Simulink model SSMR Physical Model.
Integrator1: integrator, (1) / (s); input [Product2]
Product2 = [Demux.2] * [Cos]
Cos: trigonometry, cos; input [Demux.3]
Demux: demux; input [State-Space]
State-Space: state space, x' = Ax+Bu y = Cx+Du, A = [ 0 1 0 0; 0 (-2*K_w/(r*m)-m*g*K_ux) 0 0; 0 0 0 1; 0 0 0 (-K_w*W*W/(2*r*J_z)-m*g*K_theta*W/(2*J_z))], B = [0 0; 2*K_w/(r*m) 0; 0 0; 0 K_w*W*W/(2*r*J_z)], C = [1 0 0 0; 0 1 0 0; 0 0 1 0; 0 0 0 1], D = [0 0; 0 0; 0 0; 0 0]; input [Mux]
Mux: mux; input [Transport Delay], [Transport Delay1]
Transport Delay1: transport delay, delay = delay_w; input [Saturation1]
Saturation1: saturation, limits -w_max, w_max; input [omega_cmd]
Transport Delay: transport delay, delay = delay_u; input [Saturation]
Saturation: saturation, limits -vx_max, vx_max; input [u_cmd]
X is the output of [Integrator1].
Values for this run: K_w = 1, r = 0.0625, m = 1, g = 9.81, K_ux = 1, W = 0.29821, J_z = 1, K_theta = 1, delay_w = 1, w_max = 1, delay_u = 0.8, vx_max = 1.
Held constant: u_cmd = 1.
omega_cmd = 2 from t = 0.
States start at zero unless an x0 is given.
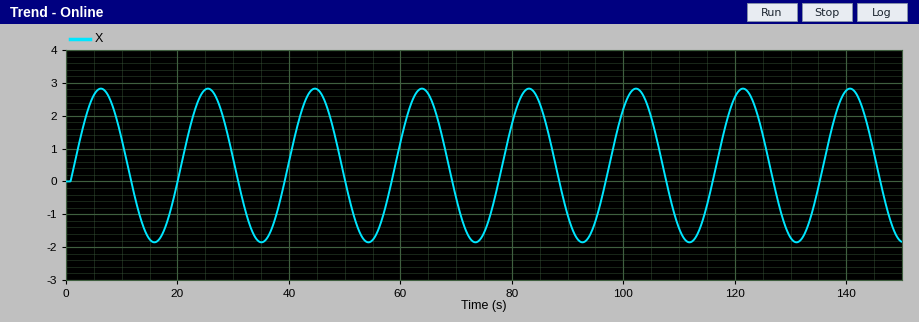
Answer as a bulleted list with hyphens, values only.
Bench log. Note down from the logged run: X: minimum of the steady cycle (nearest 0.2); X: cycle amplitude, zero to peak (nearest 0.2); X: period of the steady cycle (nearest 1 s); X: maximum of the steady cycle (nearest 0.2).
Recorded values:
- -1.8
- 2.4
- 19 s
- 2.8
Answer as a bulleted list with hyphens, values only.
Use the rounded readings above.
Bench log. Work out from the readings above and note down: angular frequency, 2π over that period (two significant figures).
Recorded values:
- 0.33 rad/s
